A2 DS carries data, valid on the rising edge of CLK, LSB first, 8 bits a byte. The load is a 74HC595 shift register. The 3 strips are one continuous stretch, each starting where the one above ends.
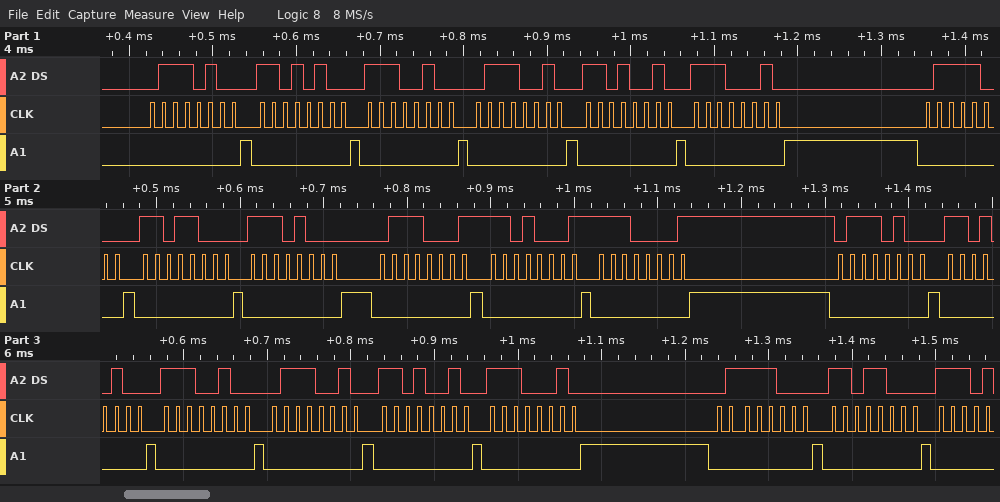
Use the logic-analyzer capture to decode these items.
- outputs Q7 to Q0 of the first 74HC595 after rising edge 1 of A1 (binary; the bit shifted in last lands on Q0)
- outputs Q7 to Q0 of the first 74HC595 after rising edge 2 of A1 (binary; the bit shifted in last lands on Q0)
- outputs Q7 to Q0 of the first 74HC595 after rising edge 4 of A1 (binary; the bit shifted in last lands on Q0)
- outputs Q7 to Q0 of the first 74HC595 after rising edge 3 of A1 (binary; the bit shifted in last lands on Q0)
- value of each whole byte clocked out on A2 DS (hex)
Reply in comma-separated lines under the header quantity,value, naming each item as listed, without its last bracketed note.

quantity,value
outputs Q7 to Q0 of the first 74HC595 after rising edge 1 of A1,01110100
outputs Q7 to Q0 of the first 74HC595 after rising edge 2 of A1,11010100
outputs Q7 to Q0 of the first 74HC595 after rising edge 4 of A1,01110010
outputs Q7 to Q0 of the first 74HC595 after rising edge 3 of A1,11100100
value of each whole byte clocked out on A2 DS,2E 2B 27 4E 4B 47 1E 1B 17 8E 8B 87 2E 2B 27 4E 4B 47 1E 1B
